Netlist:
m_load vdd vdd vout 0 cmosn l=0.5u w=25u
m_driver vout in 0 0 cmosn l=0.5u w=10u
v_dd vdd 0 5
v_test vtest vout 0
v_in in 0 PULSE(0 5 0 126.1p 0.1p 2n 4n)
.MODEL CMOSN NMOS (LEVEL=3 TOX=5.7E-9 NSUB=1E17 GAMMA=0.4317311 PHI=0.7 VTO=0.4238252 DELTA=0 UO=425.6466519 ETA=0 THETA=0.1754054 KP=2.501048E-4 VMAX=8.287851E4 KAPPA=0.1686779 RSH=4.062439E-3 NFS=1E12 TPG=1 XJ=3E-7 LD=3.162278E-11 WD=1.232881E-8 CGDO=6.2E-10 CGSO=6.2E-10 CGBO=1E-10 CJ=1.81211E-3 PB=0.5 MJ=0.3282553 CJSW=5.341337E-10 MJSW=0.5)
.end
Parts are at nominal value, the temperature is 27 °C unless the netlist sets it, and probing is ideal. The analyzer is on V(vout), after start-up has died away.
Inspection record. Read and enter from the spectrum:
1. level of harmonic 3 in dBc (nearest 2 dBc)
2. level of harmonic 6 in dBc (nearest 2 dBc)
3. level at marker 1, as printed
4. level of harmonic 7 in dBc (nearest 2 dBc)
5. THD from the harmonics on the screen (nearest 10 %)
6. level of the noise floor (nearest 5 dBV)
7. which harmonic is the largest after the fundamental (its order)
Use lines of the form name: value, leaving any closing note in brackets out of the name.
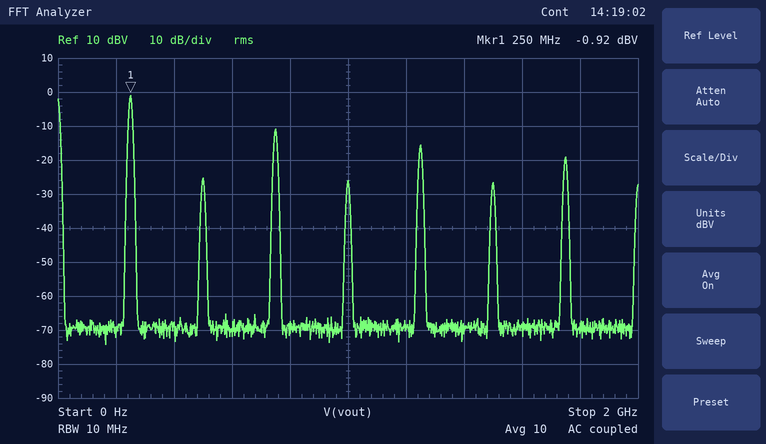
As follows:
level of harmonic 3 in dBc: -10 dBc
level of harmonic 6 in dBc: -26 dBc
level at marker 1, as printed: -0.92 dBV
level of harmonic 7 in dBc: -18 dBc
THD from the harmonics on the screen: 40 %
level of the noise floor: -70 dBV
which harmonic is the largest after the fundamental: 3
